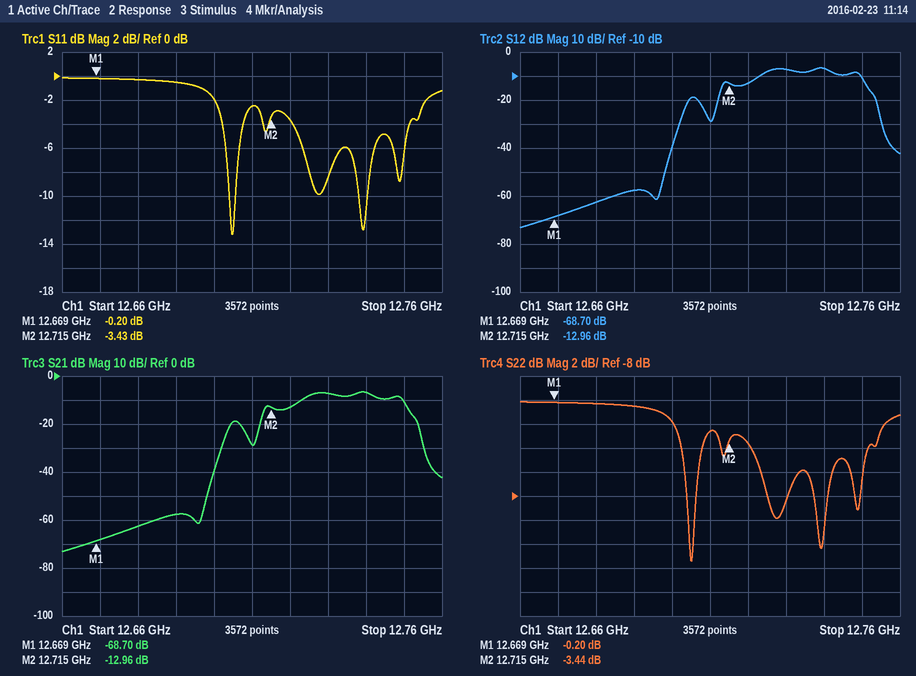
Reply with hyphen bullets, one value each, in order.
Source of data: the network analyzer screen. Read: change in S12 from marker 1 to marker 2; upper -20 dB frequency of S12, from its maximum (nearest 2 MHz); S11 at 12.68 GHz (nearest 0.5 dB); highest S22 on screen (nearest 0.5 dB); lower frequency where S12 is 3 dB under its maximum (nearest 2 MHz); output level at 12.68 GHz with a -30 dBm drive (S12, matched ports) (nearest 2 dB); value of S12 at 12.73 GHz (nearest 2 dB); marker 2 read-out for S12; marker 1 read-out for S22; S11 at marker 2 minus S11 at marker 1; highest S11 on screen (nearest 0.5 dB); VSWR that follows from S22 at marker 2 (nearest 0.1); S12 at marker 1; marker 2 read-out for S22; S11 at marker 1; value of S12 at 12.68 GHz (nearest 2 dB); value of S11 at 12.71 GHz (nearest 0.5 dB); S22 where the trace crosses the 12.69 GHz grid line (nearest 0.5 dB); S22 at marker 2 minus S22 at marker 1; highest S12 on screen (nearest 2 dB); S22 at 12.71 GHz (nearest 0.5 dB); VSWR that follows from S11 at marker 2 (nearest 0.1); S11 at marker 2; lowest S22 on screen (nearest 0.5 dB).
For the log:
- 55.74 dB
- 12.754 GHz
- -0.5 dB
- 0.0 dB
- 12.724 GHz
- -92 dBm
- -8 dB
- -12.96 dB
- -0.20 dB
- -3.23 dB
- 0.0 dB
- 5.1
- -68.70 dB
- -3.44 dB
- -0.20 dB
- -62 dB
- -2.5 dB
- -0.5 dB
- -3.24 dB
- -6 dB
- -2.5 dB
- 5.1
- -3.43 dB
- -13.5 dB
